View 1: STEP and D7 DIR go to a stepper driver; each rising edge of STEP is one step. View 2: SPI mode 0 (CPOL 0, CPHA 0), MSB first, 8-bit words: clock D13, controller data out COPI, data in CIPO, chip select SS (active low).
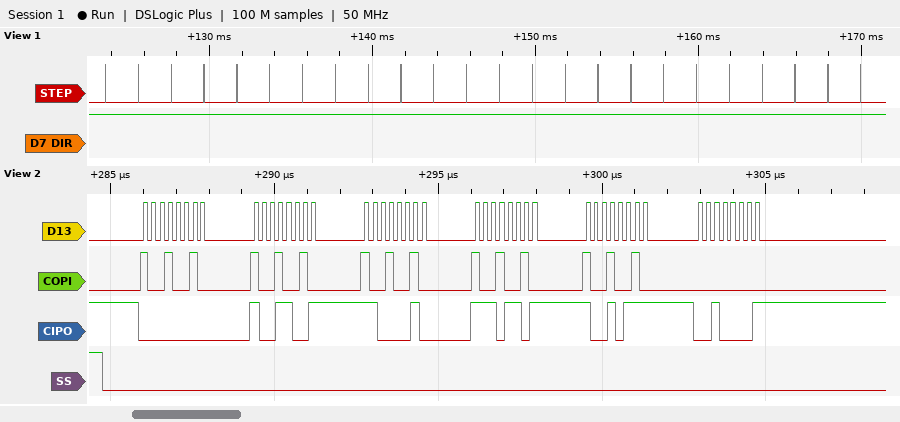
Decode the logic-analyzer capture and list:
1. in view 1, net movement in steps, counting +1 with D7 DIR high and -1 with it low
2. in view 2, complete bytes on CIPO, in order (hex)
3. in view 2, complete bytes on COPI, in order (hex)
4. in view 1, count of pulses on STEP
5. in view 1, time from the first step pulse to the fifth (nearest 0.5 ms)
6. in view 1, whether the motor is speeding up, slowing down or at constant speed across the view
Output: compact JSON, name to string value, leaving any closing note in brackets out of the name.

{"in view 1, net movement in steps, counting +1 with D7 DIR high and -1 with it low": "+24", "in view 2, complete bytes on CIPO, in order": "0x00 0x99 0xC2 0xED 0x97 0x21", "in view 2, complete bytes on COPI, in order": "0x92 0x92 0x92 0x92 0x92 0x00", "in view 1, count of pulses on STEP": "24", "in view 1, time from the first step pulse to the fifth": "8.0 ms", "in view 1, whether the motor is speeding up, slowing down or at constant speed across the view": "constant speed"}
